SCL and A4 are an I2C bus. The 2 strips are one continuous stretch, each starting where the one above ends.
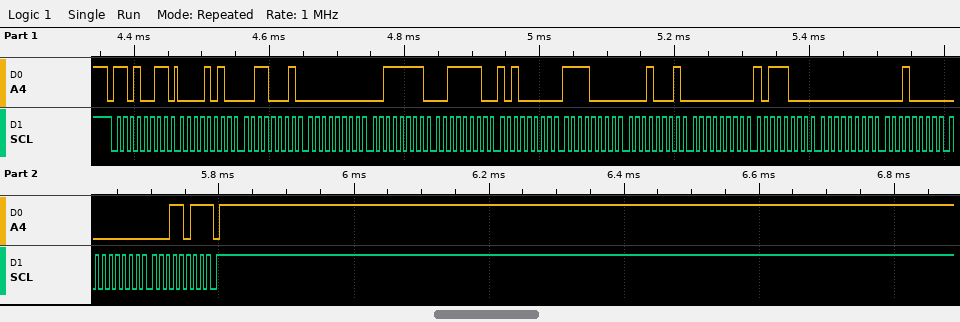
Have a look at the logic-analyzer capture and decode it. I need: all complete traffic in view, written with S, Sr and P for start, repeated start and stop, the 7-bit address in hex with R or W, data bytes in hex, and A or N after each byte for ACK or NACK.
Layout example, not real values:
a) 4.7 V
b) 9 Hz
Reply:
a) S 69R A 0A A 31 A 00 A 3F A 3E A A0 A F0 A 11 A 00 A B8 A 00 A 10 A 00 A 1B N P
